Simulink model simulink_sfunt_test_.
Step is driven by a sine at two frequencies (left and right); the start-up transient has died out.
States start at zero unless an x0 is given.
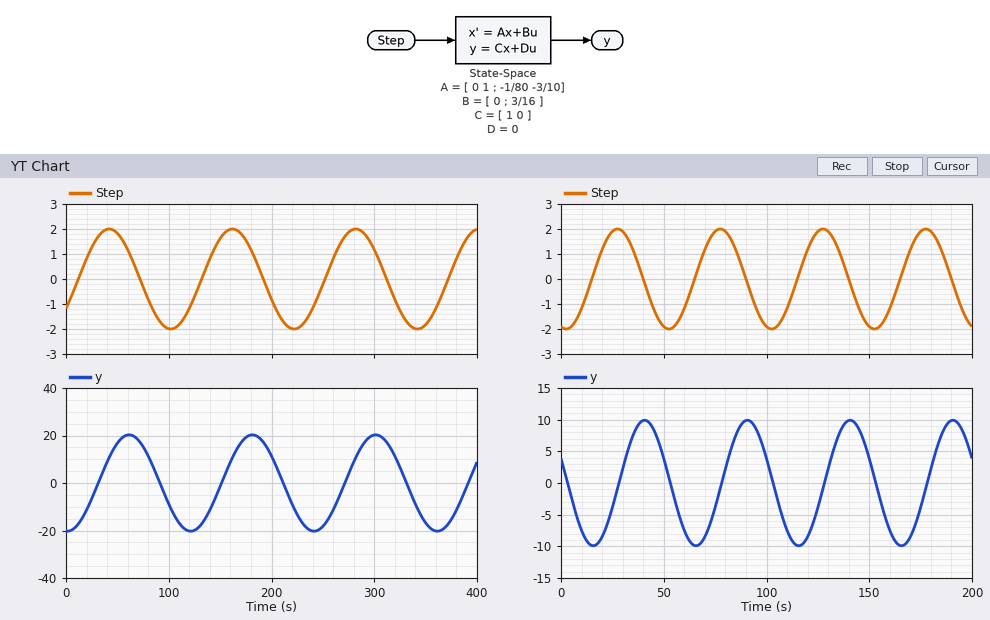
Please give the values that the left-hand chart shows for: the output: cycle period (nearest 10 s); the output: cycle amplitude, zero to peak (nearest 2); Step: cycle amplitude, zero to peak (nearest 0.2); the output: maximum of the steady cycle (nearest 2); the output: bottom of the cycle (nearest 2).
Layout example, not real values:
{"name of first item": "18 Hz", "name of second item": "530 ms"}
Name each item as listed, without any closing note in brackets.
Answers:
{"the output: cycle period": "120 s", "the output: cycle amplitude, zero to peak": "20", "Step: cycle amplitude, zero to peak": "2.0", "the output: maximum of the steady cycle": "20", "the output: bottom of the cycle": "-20"}
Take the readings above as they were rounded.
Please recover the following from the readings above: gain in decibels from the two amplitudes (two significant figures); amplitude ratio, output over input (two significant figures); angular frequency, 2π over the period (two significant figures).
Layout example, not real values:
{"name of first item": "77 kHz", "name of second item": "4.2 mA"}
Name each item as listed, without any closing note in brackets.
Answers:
{"gain in decibels from the two amplitudes": "20 dB", "amplitude ratio, output over input": "10", "angular frequency, 2π over the period": "0.052 rad/s"}
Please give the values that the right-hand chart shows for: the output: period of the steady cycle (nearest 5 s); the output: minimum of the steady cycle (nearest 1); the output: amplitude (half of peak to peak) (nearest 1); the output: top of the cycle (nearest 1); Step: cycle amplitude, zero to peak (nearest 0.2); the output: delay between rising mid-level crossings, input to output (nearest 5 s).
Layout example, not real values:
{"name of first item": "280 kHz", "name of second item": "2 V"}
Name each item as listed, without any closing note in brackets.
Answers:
{"the output: period of the steady cycle": "50 s", "the output: minimum of the steady cycle": "-10", "the output: amplitude (half of peak to peak)": "10", "the output: top of the cycle": "10", "Step: cycle amplitude, zero to peak": "2.0", "the output: delay between rising mid-level crossings, input to output": "15 s"}
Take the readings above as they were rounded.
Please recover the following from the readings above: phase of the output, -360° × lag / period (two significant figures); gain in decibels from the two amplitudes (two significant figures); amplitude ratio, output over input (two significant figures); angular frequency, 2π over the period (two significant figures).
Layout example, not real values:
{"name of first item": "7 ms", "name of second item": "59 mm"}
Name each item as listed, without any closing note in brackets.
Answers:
{"phase of the output, -360° × lag / period": "-110°", "gain in decibels from the two amplitudes": "14 dB", "amplitude ratio, output over input": "5.0", "angular frequency, 2π over the period": "0.13 rad/s"}
